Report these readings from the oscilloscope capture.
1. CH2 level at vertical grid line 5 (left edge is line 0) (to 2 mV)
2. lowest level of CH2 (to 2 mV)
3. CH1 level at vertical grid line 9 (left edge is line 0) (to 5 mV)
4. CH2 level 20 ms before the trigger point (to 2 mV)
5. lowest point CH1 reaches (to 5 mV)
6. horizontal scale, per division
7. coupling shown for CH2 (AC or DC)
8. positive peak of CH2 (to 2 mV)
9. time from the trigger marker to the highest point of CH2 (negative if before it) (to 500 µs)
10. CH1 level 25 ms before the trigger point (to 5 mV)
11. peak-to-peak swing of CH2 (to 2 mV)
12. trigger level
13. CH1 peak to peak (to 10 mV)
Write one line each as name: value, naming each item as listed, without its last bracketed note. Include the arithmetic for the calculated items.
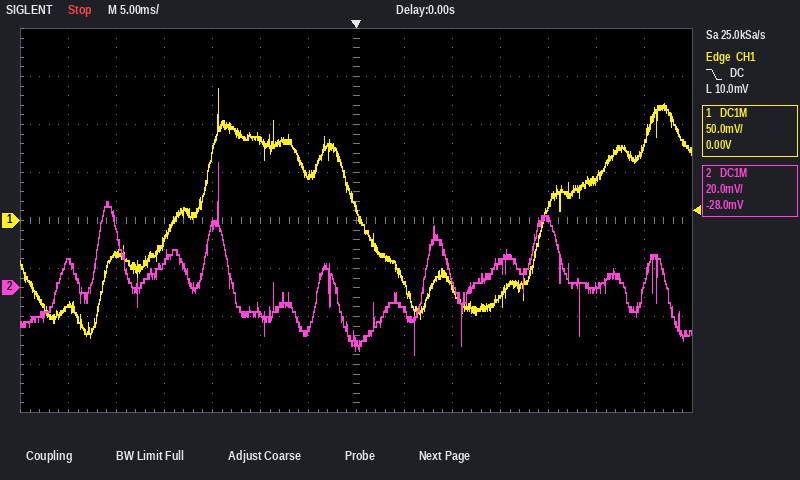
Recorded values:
CH2 level at vertical grid line 5 (left edge is line 0): -10 mV
lowest level of CH2: -28 mV
CH1 level at vertical grid line 9 (left edge is line 0): -70 mV
CH2 level 20 ms before the trigger point: 10 mV
lowest point CH1 reaches: -120 mV
horizontal scale, per division: 5 ms
coupling shown for CH2: DC
positive peak of CH2: 52 mV
time from the trigger marker to the highest point of CH2 (negative if before it): -14.5 ms
CH1 level 25 ms before the trigger point: -35 mV
peak-to-peak swing of CH2: 52 mV − (-28 mV) = 80 mV
trigger level: 10.0 mV
CH1 peak to peak: 260 mV
